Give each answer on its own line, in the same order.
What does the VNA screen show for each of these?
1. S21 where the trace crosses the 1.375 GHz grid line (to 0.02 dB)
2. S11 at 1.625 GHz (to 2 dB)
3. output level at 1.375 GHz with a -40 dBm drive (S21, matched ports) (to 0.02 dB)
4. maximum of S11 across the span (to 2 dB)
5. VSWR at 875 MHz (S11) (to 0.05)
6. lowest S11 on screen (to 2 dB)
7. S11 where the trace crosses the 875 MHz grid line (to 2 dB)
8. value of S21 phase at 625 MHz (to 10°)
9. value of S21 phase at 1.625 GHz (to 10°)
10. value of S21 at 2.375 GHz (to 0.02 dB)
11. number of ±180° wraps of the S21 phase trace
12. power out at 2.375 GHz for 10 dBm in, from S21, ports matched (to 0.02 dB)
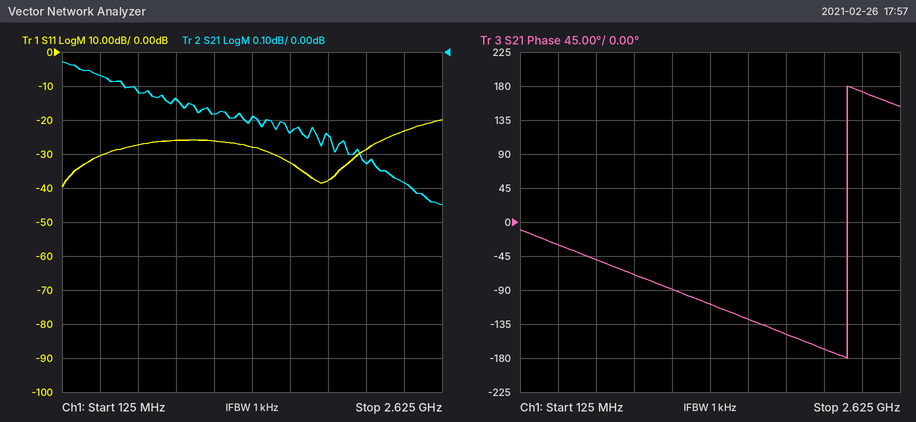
-0.20 dB
-32 dB
-40.20 dBm
-20 dB
1.10
-40 dB
-26 dB
-50°
-130°
-0.38 dB
1
9.62 dBm
